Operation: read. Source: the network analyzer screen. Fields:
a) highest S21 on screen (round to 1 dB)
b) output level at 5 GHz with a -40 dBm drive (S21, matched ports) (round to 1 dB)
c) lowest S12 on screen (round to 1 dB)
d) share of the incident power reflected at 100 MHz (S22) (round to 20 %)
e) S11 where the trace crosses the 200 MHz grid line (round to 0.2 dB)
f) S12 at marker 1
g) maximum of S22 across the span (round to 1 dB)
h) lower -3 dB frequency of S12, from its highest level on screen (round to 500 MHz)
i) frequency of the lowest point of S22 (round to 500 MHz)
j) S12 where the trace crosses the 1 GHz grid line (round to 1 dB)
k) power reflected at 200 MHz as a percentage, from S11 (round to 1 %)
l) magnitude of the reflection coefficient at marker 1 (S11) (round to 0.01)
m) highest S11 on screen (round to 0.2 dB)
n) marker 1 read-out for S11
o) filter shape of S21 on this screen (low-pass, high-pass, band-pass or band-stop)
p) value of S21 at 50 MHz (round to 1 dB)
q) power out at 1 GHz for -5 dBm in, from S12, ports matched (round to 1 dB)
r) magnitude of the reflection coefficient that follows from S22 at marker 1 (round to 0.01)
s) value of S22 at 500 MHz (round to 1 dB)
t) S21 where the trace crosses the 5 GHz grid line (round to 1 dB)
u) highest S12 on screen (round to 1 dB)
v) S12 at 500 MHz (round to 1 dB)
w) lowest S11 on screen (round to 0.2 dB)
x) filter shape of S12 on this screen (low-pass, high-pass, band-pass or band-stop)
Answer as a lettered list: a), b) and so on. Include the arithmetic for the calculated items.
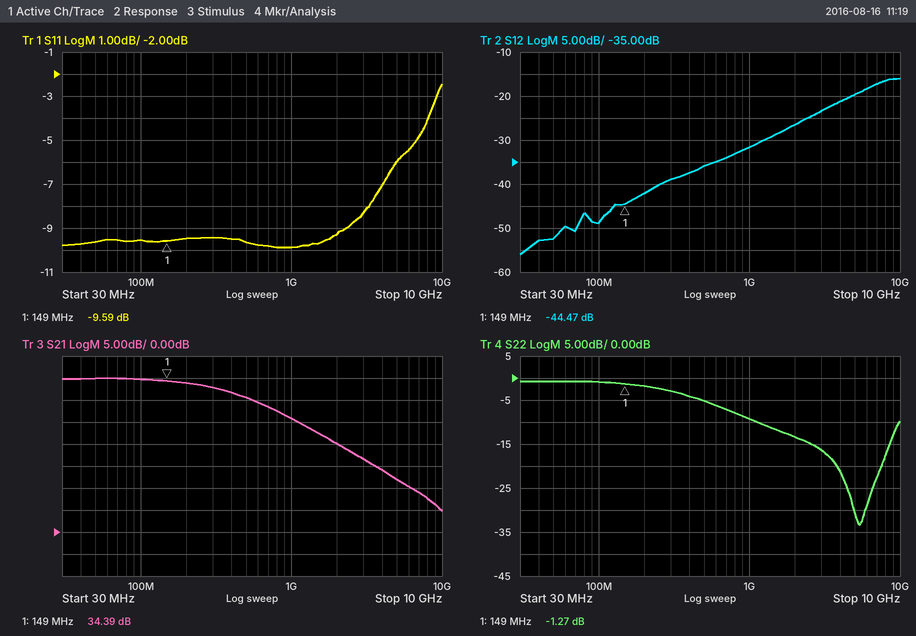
a) 35 dB
b) -40 dBm + (12 dB) = -28 dBm
c) -56 dB
d) 10^(-1/10) ≈ 79.4 %, so 80 % to the nearest 20 %
e) -9.4 dB
f) -44.47 dB
g) -1 dB
h) 5.5 GHz
i) 5.5 GHz
j) -32 dB
k) 10^(-9.4/10) ≈ 11 %
l) 10^(-9.59/20) ≈ 0.33
m) -2.4 dB
n) -9.59 dB
o) low-pass
p) 35 dB
q) -5 dBm + (-32 dB) = -37 dBm
r) 10^(-1.27/20) ≈ 0.86
s) -5 dB
t) 12 dB
u) -16 dB
v) -36 dB
w) -9.8 dB
x) high-pass
